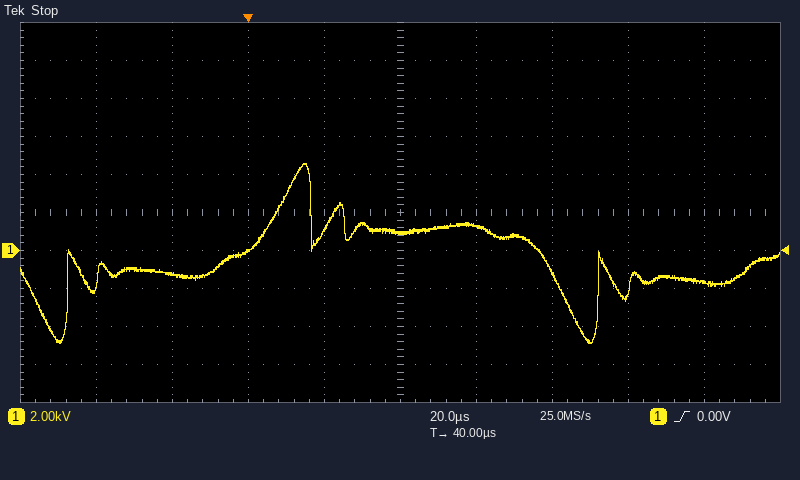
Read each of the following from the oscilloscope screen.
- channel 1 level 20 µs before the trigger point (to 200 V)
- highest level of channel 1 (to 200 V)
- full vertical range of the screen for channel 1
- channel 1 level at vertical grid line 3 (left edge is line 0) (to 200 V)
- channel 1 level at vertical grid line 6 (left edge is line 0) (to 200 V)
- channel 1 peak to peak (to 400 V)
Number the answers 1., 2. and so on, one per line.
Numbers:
1. -1.2 kV
2. 4.6 kV
3. 20 kV
4. 0.0 kV
5. 1.2 kV
6. 9.6 kV
